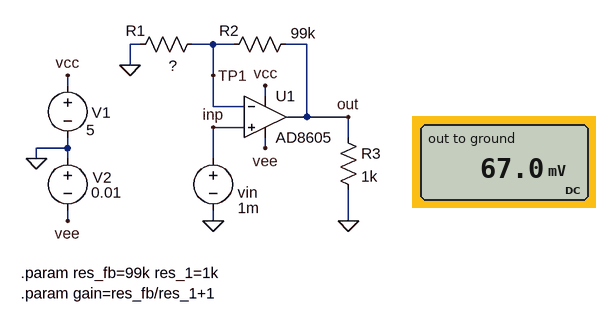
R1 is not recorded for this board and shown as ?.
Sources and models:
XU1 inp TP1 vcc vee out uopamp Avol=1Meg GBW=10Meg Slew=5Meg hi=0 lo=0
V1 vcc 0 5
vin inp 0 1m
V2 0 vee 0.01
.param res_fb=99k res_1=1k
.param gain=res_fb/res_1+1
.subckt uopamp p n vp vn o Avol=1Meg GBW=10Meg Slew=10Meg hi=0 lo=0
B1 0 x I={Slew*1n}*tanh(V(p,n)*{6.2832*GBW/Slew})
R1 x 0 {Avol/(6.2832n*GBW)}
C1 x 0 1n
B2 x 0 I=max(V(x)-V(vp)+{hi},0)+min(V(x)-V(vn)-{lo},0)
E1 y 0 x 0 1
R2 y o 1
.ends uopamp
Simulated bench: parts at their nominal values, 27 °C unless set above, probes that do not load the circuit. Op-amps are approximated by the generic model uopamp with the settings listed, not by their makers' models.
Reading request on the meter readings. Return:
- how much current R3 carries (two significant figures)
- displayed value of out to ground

67 µA
67.0 mV
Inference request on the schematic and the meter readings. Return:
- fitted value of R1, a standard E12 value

1.5 kΩ
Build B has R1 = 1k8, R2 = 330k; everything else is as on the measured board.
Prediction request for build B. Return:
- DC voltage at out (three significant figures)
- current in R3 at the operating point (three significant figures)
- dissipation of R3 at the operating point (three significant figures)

184 mV
184 µA
34.0 µW
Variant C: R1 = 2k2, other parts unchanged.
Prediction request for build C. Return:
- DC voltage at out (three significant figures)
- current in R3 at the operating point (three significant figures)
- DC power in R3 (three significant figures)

46.0 mV
46.0 µA
2.12 µW
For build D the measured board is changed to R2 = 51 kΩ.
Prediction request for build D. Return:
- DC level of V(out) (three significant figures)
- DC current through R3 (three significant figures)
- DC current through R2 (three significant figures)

35.0 mV
35.0 µA
667 nA
